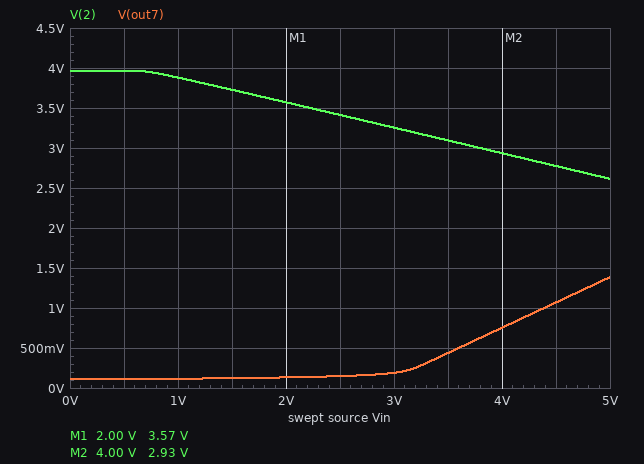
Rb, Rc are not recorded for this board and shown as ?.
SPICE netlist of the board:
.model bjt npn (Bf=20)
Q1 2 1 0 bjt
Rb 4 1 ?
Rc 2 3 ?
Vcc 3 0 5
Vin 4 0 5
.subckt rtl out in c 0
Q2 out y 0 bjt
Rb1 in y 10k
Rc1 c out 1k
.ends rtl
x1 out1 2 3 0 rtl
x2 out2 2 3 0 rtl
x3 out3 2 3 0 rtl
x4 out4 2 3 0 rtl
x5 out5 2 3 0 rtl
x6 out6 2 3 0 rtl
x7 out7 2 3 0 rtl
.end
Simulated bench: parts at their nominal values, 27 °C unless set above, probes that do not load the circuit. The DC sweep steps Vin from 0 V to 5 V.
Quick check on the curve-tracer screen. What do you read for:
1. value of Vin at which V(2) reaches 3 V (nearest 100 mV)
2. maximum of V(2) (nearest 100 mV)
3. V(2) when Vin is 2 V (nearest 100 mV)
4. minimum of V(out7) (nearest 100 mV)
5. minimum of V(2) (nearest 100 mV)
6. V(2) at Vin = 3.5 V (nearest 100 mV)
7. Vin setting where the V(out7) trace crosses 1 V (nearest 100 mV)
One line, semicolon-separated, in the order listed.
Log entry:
3.8 V; 4.0 V; 3.6 V; 100 mV; 2.6 V; 3.1 V; 4.4 V
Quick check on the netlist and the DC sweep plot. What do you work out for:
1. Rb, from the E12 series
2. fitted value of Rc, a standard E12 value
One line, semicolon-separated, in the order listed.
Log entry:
22 kΩ; 470 Ω
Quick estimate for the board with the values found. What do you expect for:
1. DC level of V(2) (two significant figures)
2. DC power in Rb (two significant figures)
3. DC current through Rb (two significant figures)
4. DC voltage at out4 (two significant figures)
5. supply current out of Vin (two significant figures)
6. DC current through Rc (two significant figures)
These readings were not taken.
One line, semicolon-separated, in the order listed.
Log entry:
2.6 V; 800 µW; 190 µA; 1.4 V; 190 µA; 5.1 mA
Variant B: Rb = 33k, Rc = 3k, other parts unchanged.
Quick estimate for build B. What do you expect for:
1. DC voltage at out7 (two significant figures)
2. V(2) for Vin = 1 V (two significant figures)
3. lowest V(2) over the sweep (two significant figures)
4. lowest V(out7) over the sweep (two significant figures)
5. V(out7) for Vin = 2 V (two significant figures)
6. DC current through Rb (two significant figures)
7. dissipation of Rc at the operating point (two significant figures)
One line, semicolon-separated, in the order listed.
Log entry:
5.0 V; 2.0 V; 96 mV; 2.3 V; 3.7 V; 130 µA; 8.0 mW
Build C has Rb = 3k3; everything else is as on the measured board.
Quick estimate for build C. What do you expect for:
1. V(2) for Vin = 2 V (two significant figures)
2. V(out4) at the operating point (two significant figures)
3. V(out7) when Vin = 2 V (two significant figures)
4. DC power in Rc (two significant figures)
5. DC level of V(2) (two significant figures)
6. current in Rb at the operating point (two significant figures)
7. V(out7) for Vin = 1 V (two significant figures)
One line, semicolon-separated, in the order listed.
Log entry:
1.4 V; 5.0 V; 3.7 V; 52 mW; 74 mV; 1.3 mA; 140 mV
